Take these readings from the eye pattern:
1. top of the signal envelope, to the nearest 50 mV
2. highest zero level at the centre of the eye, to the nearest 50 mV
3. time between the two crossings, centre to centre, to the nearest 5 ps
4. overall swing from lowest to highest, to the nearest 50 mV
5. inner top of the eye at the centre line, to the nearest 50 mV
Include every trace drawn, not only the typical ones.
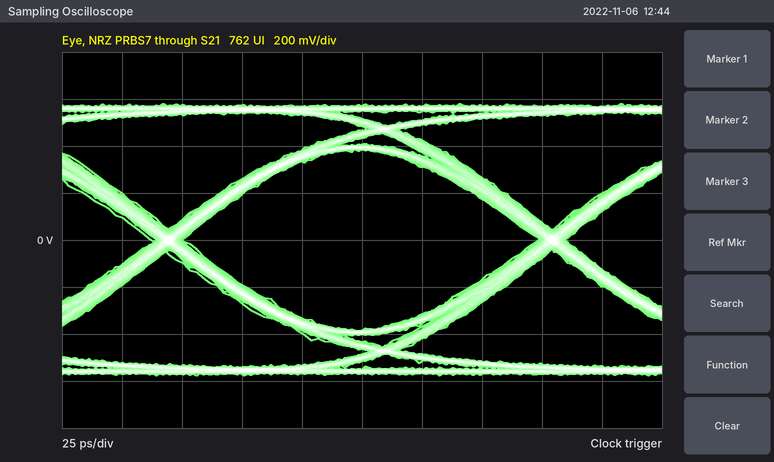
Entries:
600 mV
-400 mV
160 ps
1.15 V
400 mV
